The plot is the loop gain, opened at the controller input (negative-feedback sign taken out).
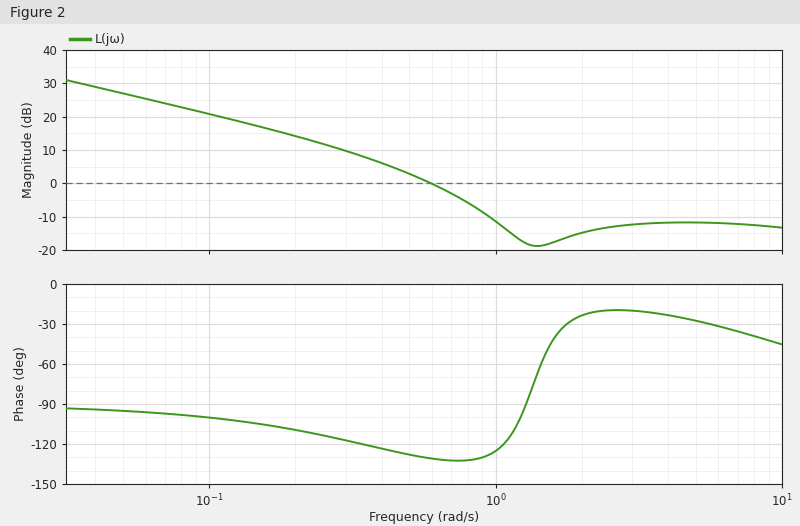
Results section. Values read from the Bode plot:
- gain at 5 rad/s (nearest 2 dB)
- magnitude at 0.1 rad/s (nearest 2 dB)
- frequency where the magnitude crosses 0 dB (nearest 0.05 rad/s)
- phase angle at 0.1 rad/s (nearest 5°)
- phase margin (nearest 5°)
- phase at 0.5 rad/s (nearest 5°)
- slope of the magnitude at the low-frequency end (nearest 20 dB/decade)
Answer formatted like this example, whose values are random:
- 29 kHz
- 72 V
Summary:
- -12 dB
- 20 dB
- 0.60 rad/s
- -100°
- 50°
- -130°
- -20 dB/decade
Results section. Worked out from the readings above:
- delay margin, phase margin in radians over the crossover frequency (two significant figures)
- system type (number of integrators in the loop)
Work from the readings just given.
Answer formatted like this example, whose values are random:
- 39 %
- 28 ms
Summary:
- 1.5 s
- 1
